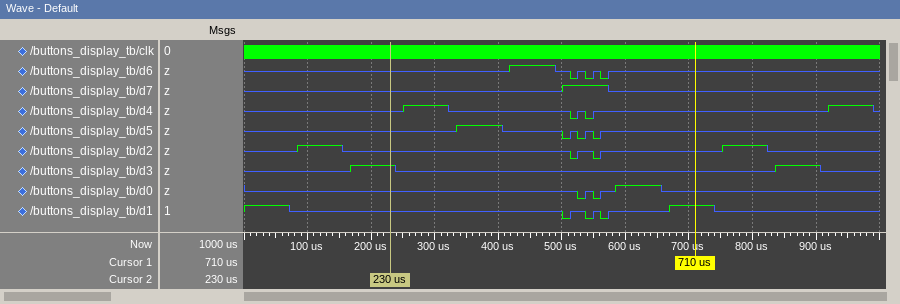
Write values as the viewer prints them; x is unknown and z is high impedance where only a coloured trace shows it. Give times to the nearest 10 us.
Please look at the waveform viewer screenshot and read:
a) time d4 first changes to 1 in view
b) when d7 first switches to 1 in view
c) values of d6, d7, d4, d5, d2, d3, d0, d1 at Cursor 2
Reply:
250 us
500 us
d6=z, d7=z, d4=z, d5=z, d2=z, d3=1, d0=z, d1=z
